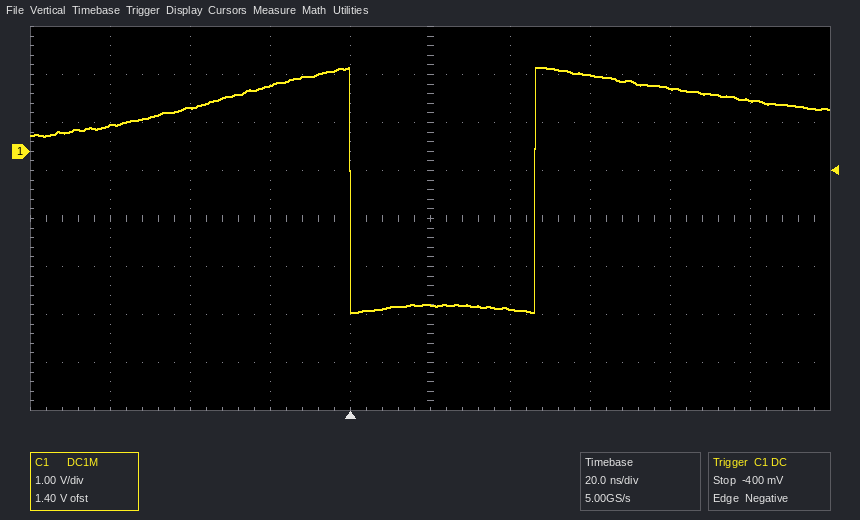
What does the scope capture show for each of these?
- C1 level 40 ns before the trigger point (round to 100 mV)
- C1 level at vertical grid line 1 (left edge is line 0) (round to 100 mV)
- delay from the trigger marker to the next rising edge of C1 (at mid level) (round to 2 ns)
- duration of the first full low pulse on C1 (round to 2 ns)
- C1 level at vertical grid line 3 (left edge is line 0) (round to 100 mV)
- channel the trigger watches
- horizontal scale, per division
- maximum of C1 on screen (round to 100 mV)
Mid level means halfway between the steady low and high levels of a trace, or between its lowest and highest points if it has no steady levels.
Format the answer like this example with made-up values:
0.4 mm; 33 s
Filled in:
900 mV; 500 mV; 46 ns; 46 ns; 1.4 V; C1; 20 ns; 1.7 V
